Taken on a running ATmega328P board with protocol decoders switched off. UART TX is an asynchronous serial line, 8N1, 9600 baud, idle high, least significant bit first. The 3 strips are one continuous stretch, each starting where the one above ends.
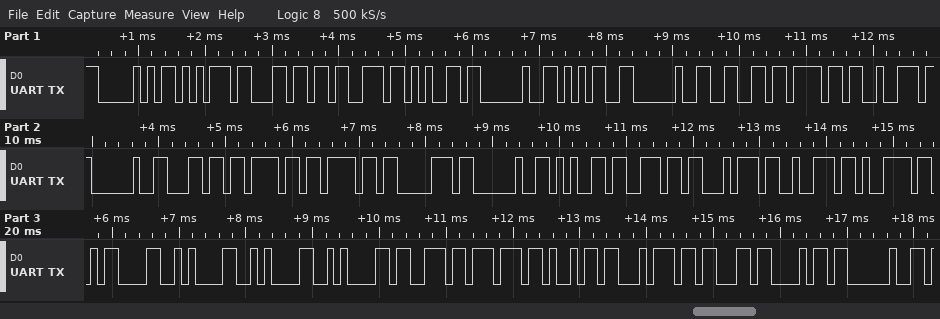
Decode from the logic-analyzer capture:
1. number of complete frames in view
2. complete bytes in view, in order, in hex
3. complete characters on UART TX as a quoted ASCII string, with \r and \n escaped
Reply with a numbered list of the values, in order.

1. 33
2. 50 75 6C 73 65 20 35 20 66 6F 72 20 6C 6F 6F 70 20 65 6E 74 72 79 0D 0A 0A 0A 73 77 69 74 63 68 20
3. "Pulse 5 for loop entry\r\n\n\nswitch "
